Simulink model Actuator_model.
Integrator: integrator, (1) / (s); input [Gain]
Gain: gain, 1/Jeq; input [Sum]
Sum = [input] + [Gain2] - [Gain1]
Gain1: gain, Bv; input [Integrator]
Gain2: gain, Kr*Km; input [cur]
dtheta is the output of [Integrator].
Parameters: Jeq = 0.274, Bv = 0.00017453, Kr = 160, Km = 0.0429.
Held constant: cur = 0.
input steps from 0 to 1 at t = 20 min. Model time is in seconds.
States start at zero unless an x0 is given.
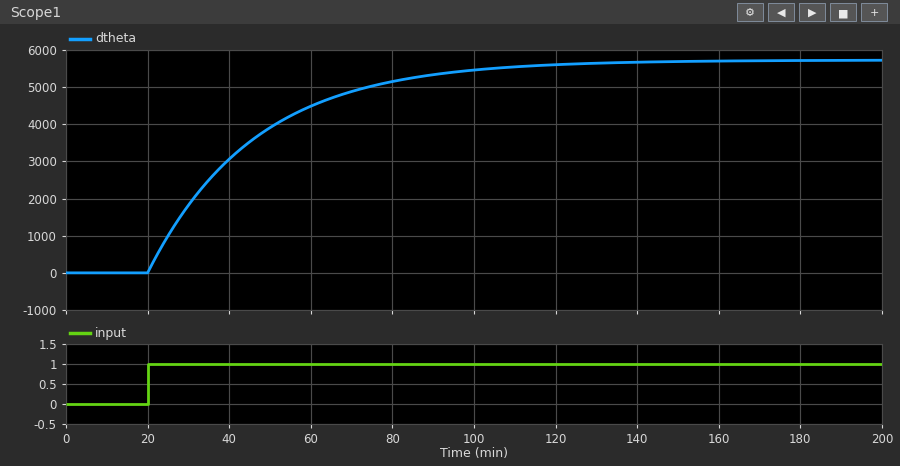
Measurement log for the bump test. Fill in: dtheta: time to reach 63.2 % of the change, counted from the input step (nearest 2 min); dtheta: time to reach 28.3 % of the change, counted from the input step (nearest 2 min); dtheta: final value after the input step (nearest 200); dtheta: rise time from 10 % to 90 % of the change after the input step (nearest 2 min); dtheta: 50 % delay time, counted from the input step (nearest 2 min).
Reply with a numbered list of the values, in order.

1. 26 min
2. 8 min
3. 5800
4. 58 min
5. 18 min
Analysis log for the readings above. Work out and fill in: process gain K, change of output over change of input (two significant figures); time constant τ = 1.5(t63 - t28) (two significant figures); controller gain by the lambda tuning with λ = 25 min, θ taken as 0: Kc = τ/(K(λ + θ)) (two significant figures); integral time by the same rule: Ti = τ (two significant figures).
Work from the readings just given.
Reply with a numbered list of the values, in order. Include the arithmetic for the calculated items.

1. (5800 - 0) / 1 = 5800
2. 1.5 × (26 - 8) = 27 min
3. 27 / (5800 × (25 + 0)) = 0.00019
4. 27 min
